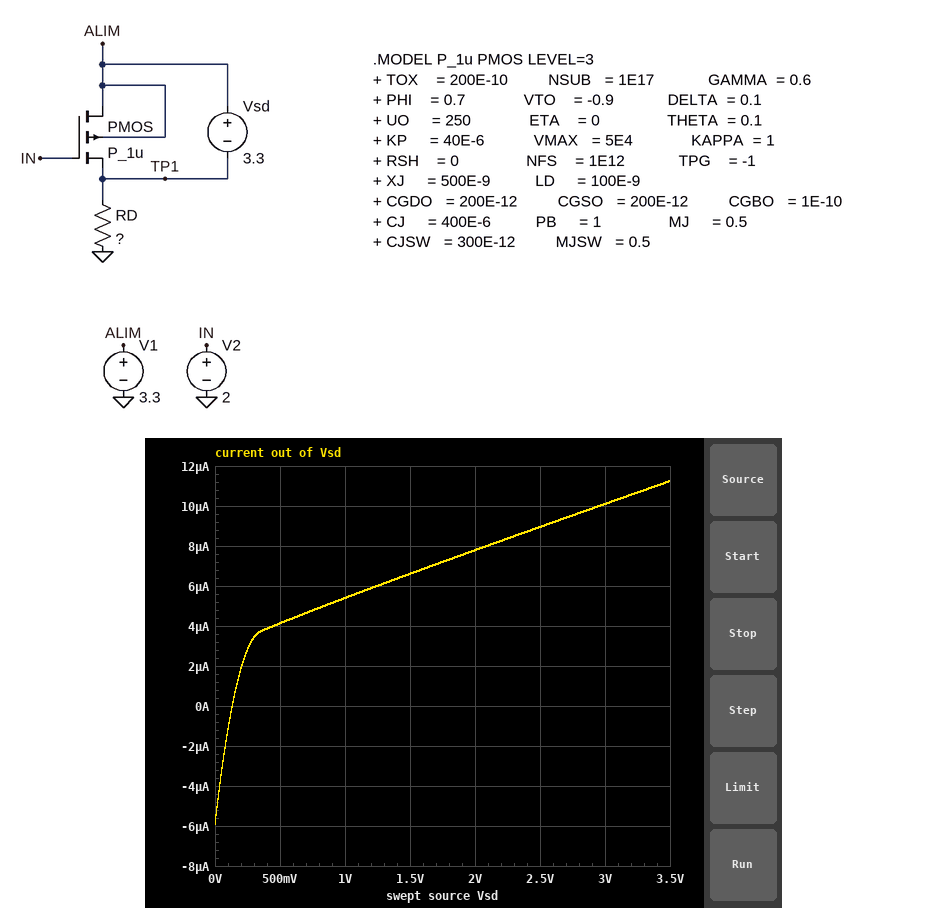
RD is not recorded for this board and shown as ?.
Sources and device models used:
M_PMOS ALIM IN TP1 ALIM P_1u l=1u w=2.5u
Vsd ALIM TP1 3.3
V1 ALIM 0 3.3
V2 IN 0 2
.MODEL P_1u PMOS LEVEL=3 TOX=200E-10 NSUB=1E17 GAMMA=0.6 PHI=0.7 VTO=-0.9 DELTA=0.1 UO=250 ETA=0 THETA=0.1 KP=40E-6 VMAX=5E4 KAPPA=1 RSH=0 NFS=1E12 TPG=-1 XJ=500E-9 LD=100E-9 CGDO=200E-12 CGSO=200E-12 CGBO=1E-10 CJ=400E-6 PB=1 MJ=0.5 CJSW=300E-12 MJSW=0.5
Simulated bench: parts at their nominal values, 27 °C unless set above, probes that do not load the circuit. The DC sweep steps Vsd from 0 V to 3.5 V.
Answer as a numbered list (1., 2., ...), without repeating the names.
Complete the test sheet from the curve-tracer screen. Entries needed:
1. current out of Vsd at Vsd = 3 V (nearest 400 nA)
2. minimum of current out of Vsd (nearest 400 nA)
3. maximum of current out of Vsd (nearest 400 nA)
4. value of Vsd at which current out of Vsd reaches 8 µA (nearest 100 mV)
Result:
1. 10.0 µA
2. -6.0 µA
3. 11.2 µA
4. 2.1 V
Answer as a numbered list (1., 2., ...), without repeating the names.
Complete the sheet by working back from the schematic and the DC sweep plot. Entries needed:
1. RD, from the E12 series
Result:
1. 560 kΩ
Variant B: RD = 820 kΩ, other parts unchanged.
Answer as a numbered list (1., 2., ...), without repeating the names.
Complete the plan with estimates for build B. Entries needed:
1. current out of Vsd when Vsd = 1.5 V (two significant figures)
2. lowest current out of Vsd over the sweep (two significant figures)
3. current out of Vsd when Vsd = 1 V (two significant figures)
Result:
1. 7.6 µA
2. -4.0 µA
3. 6.7 µA
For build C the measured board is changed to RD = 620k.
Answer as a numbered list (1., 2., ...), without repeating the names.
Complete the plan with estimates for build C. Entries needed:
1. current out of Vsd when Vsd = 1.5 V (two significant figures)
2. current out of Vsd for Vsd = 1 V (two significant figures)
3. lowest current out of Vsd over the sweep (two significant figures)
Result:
1. 6.9 µA
2. 5.8 µA
3. -5.3 µA
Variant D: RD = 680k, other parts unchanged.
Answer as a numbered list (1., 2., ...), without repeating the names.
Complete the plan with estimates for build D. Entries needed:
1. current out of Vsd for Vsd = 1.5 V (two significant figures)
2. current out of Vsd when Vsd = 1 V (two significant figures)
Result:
1. 7.2 µA
2. 6.1 µA
